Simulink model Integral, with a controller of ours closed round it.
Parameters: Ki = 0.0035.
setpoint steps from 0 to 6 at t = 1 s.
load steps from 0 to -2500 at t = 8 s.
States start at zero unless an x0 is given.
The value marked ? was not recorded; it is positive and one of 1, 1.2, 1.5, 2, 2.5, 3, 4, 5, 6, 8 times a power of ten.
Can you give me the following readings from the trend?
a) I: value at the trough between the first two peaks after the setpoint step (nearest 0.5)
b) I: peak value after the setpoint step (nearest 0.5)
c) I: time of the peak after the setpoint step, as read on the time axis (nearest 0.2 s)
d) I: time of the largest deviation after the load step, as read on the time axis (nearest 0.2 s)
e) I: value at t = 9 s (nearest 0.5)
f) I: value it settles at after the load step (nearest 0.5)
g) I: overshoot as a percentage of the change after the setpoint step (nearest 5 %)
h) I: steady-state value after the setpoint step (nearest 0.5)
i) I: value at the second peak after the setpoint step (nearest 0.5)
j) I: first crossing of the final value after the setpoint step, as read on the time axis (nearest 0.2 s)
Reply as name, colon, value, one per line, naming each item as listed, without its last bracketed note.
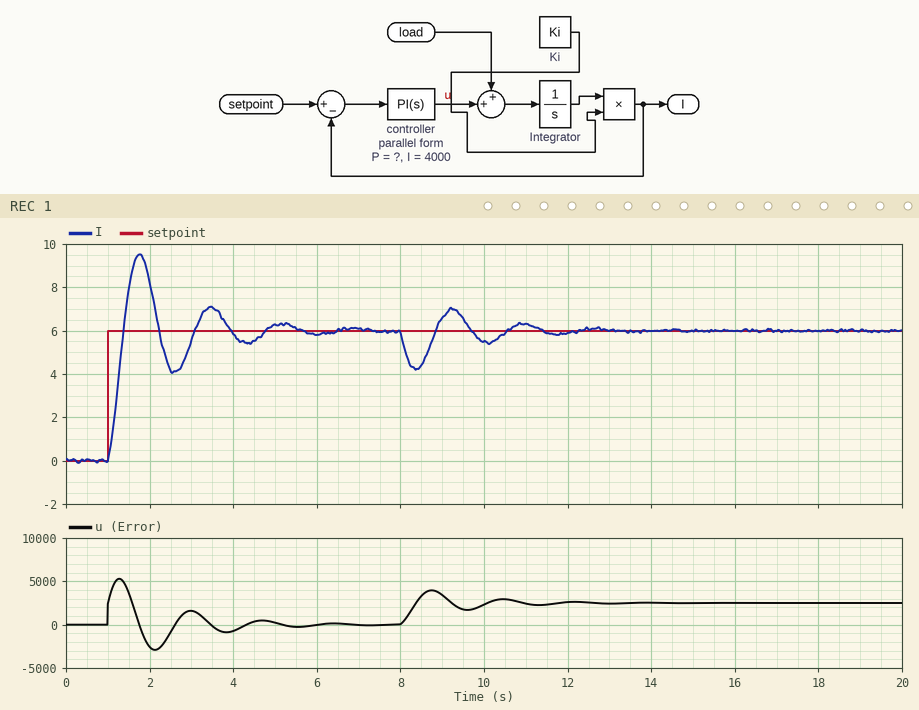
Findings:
I: value at the trough between the first two peaks after the setpoint step: 4.0
I: peak value after the setpoint step: 9.5
I: time of the peak after the setpoint step, as read on the time axis: 1.8 s
I: time of the largest deviation after the load step, as read on the time axis: 8.4 s
I: value at t = 9 s: 6.5
I: value it settles at after the load step: 6.0
I: overshoot as a percentage of the change after the setpoint step: 60 %
I: steady-state value after the setpoint step: 6.0
I: value at the second peak after the setpoint step: 7.0
I: first crossing of the final value after the setpoint step, as read on the time axis: 1.4 s
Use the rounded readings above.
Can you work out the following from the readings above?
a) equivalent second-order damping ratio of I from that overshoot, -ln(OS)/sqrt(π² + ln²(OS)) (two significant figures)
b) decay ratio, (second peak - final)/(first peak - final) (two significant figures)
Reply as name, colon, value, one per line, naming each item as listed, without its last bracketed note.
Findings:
equivalent second-order damping ratio of I from that overshoot, -ln(OS)/sqrt(π² + ln²(OS)): 0.16
decay ratio, (second peak - final)/(first peak - final): 0.29
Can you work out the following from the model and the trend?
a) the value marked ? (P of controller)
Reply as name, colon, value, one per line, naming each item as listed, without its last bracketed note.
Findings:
the value marked ?: 400
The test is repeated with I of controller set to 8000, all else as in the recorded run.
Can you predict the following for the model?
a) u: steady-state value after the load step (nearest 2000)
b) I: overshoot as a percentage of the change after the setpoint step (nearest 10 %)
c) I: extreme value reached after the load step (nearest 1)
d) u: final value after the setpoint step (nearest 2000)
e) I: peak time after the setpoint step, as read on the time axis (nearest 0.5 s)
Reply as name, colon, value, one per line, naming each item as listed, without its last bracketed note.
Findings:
u: steady-state value after the load step: 2000
I: overshoot as a percentage of the change after the setpoint step: 70 %
I: extreme value reached after the load step: 5
u: final value after the setpoint step: 0
I: peak time after the setpoint step, as read on the time axis: 1.5 s
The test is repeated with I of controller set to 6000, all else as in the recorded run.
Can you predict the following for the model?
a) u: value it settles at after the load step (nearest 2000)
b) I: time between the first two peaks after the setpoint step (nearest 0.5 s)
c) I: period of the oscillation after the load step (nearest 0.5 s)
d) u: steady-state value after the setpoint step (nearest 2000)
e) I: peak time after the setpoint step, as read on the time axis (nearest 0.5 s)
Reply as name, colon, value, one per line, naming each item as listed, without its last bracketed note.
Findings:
u: value it settles at after the load step: 2000
I: time between the first two peaks after the setpoint step: 1.5 s
I: period of the oscillation after the load step: 1.5 s
u: steady-state value after the setpoint step: 0
I: peak time after the setpoint step, as read on the time axis: 1.5 s
